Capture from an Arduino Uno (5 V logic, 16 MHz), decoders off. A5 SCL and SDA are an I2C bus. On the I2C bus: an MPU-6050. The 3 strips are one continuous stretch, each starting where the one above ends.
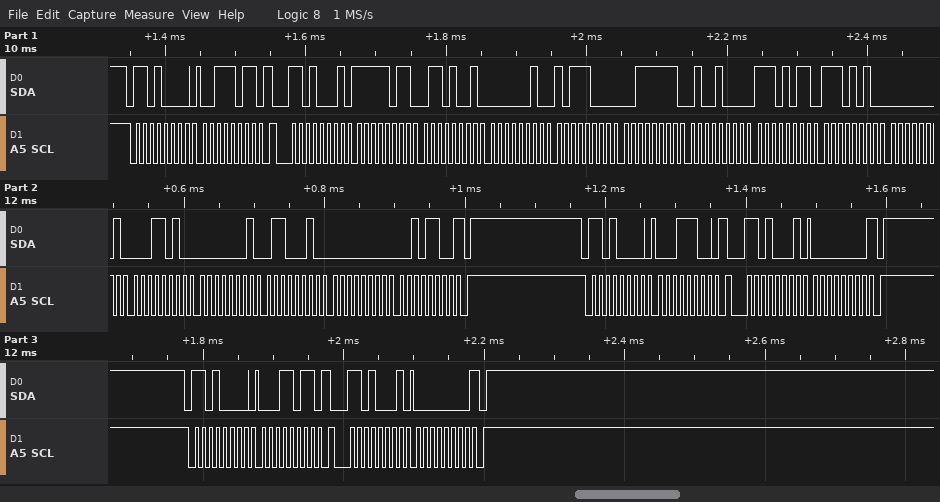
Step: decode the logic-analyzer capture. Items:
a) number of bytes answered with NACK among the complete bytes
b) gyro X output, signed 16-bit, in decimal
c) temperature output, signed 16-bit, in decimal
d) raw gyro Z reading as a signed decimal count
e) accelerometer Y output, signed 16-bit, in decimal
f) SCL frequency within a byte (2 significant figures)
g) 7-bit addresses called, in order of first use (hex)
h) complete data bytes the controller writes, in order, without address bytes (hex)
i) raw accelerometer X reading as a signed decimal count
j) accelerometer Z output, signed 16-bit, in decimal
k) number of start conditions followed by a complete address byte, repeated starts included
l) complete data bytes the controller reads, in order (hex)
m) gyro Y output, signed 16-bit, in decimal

3
282
-5142
44
696
100 kHz
0x68
3B 1C 1B
-1175
16200
6
FB 69 02 B8 3F 48 EB EA 01 1A 01 62 00 2C 00 00
354
